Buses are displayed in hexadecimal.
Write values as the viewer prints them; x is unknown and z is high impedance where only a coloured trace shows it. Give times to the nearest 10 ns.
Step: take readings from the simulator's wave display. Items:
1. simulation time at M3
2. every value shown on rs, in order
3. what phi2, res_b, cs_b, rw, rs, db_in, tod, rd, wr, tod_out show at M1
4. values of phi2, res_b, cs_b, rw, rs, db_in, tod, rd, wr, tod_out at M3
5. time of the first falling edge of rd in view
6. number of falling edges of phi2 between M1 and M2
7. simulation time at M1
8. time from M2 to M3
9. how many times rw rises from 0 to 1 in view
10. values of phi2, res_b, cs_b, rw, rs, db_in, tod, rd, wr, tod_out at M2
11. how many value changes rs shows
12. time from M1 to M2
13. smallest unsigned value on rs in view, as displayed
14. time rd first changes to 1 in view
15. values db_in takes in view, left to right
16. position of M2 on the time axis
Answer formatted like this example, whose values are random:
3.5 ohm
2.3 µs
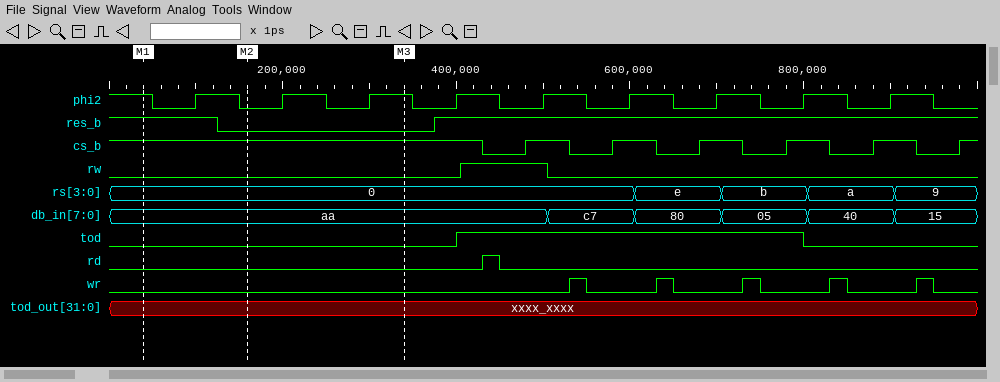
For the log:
340 ns
0, e, b, a, 9
phi2=1, res_b=1, cs_b=1, rw=0, rs=0, db_in=aa, tod=0, rd=0, wr=0, tod_out=xxxx_xxxx
phi2=1, res_b=0, cs_b=1, rw=0, rs=0, db_in=aa, tod=0, rd=0, wr=0, tod_out=xxxx_xxxx
450 ns
2
40 ns
180 ns
1
phi2=0, res_b=0, cs_b=1, rw=0, rs=0, db_in=aa, tod=0, rd=0, wr=0, tod_out=xxxx_xxxx
4
120 ns
0
430 ns
aa, c7, 80, 05, 40, 15
160 ns
